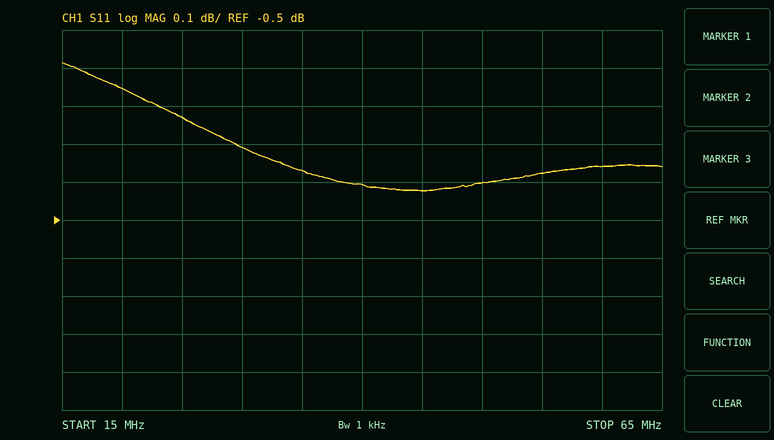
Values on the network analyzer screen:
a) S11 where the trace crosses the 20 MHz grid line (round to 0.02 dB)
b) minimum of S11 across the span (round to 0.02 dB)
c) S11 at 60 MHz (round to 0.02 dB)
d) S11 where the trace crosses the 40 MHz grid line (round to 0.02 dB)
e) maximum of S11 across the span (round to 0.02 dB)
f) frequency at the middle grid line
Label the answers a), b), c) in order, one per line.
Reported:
a) -0.16 dB
b) -0.42 dB
c) -0.36 dB
d) -0.40 dB
e) -0.08 dB
f) 40 MHz
